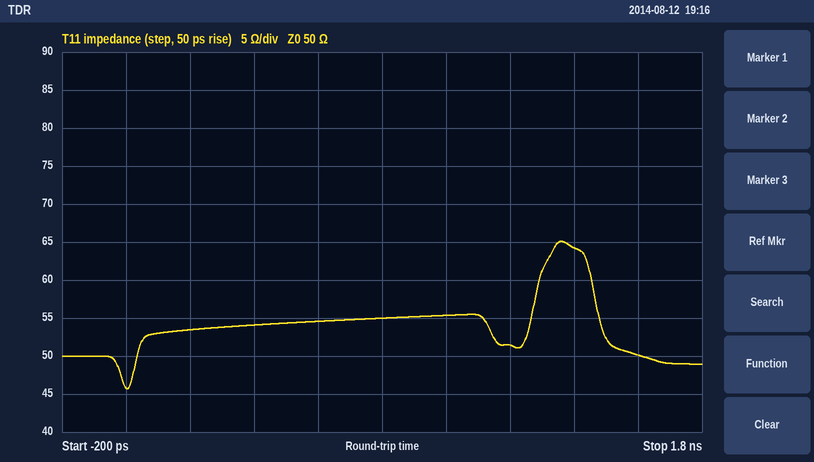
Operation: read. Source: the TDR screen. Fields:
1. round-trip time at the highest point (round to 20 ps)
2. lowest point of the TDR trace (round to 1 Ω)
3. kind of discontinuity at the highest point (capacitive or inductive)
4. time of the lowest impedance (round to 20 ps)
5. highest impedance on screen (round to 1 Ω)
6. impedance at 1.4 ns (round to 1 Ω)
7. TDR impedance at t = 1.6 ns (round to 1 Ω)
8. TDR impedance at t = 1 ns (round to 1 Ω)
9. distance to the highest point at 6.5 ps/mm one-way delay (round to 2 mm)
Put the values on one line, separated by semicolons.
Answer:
1.36 ns; 46 Ω; inductive; 0 ps; 65 Ω; 64 Ω; 50 Ω; 55 Ω; 104 mm
